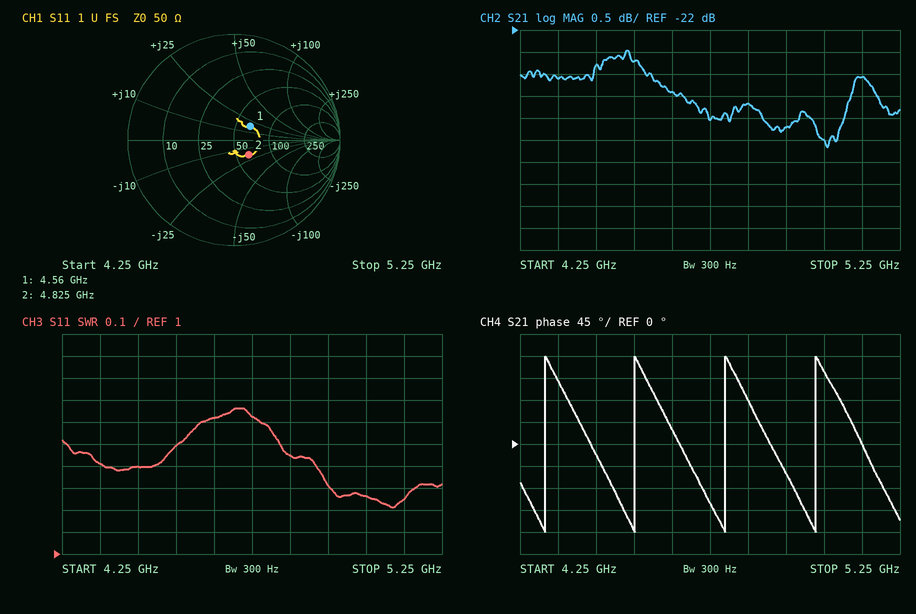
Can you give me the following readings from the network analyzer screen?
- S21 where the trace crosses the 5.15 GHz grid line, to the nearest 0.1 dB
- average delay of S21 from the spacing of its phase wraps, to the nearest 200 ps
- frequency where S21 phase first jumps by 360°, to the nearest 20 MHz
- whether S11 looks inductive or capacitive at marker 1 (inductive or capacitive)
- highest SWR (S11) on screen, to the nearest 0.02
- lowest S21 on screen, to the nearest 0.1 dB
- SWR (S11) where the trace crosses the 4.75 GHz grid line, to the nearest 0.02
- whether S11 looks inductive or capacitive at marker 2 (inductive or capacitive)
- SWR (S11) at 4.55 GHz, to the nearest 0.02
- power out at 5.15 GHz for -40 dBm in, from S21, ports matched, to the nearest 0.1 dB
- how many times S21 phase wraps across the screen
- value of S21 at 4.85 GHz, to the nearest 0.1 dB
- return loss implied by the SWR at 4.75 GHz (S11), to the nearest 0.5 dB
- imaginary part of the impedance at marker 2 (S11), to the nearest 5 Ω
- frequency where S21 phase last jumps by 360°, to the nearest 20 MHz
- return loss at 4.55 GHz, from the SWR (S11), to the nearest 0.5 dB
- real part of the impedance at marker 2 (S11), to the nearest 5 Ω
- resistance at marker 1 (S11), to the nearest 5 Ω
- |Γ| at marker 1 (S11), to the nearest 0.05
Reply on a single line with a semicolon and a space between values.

-23.1 dB; 4.2 ns; 4.32 GHz; inductive; 1.66; -24.7 dB; 1.62; capacitive; 1.50; -63.1 dBm; 4; -23.7 dB; 12.5 dB; -20 Ω; 5.02 GHz; 14.0 dB; 65 Ω; 65 Ω; 0.20
